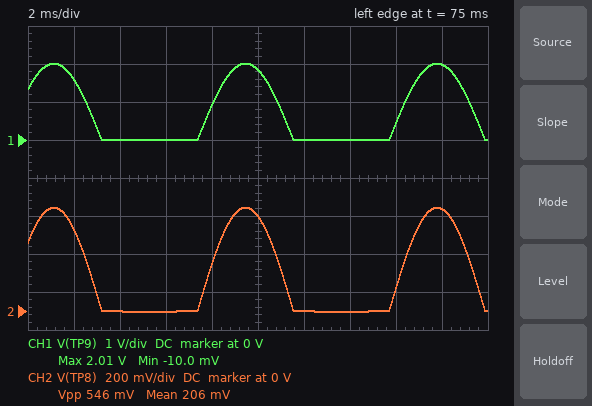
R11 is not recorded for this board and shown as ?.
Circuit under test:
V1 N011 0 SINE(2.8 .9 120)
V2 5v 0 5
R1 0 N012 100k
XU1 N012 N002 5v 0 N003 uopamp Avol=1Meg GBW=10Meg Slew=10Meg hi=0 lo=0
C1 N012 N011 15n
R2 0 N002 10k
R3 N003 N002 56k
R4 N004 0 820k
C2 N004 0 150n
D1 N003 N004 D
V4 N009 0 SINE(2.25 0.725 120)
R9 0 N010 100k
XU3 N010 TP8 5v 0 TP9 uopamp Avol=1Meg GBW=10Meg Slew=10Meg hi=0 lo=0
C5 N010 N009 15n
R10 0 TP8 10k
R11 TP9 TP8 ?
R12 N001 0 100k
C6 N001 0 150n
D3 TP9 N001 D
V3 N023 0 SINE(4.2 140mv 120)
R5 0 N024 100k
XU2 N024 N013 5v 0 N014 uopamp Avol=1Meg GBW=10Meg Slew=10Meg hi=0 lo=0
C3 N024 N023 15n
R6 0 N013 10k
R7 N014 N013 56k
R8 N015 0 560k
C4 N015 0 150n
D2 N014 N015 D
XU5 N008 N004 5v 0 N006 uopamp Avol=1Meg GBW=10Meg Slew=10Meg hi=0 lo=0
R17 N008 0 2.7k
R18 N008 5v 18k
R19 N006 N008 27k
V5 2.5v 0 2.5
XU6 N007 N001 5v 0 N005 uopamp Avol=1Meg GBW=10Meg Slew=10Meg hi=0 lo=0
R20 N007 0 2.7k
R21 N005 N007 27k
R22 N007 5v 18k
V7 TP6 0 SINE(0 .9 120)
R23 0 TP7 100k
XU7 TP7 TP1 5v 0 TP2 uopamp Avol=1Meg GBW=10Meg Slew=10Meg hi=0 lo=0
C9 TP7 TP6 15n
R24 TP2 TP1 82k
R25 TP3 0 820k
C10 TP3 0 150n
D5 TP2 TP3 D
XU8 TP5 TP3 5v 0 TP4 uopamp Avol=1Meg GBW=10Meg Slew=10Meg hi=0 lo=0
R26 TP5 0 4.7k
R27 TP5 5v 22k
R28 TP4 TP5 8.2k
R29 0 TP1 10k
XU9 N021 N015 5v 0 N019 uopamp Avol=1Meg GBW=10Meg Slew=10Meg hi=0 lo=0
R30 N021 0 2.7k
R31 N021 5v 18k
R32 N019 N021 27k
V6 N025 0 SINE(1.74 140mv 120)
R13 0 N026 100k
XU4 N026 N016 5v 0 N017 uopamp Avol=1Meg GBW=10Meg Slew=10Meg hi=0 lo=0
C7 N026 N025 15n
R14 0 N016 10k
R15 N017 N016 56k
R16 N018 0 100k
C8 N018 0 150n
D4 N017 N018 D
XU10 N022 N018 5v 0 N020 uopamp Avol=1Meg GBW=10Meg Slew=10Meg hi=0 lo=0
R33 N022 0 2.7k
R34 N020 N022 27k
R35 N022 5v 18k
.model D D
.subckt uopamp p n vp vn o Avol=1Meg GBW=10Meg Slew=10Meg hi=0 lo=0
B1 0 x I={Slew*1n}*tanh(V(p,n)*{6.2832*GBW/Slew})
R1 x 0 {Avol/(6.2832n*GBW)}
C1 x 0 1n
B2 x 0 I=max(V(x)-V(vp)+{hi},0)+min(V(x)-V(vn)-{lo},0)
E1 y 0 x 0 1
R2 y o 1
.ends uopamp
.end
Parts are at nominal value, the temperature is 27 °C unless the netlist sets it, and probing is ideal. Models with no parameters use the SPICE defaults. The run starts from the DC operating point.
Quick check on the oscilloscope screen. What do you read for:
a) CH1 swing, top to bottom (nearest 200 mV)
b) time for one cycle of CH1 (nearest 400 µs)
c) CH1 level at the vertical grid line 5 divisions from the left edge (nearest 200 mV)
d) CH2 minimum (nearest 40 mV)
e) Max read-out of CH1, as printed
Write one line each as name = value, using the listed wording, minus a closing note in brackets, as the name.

CH1 swing, top to bottom = 2.0 V
time for one cycle of CH1 = 8.4 ms
CH1 level at the vertical grid line 5 divisions from the left edge = 1.8 V
CH2 minimum = 0 V
Max read-out of CH1, as printed = 2.01 V
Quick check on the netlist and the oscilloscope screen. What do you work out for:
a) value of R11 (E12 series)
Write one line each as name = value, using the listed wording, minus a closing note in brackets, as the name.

value of R11 = 27 kΩ
